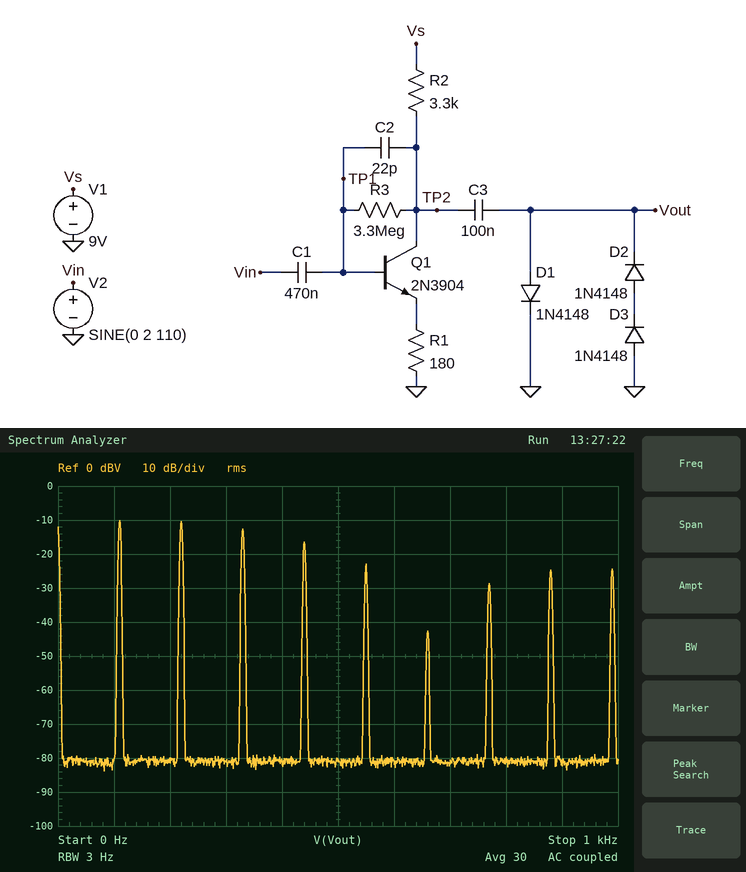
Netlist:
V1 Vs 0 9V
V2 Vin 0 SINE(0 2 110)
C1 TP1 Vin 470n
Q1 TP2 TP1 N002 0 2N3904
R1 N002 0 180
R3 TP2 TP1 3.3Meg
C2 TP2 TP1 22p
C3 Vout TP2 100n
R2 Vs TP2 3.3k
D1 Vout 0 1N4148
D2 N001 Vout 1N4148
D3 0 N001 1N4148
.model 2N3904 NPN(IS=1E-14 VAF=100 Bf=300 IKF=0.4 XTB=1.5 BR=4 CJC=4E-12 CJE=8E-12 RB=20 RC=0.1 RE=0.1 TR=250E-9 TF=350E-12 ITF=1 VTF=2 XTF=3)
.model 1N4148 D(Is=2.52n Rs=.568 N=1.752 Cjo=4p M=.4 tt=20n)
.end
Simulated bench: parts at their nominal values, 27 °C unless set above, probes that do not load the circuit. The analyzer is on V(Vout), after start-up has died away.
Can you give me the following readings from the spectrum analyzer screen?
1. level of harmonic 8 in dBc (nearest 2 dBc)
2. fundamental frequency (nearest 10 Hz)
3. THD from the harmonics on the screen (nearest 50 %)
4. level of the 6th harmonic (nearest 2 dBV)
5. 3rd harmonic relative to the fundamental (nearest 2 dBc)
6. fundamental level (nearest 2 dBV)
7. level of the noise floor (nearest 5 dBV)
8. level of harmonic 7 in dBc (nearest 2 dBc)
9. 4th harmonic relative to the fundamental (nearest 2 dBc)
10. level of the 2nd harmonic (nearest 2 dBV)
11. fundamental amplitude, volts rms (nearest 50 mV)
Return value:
-14 dBc
110 Hz
150 %
-42 dBV
-2 dBc
-10 dBV
-80 dBV
-18 dBc
-6 dBc
-10 dBV
300 mV
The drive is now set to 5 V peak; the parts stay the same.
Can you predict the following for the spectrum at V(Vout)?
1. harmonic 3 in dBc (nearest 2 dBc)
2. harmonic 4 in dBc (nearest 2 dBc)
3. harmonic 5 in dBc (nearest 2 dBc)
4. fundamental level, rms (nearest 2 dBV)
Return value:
0 dBc
-2 dBc
-4 dBc
-14 dBV
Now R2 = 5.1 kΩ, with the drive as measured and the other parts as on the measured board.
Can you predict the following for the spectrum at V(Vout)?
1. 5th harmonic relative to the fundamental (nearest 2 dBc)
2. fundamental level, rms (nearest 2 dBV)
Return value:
-10 dBc
-10 dBV
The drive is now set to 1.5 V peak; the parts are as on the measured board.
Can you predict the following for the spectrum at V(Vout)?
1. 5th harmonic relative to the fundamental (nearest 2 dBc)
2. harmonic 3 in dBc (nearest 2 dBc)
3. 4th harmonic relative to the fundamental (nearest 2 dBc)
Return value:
-22 dBc
-4 dBc
-10 dBc
